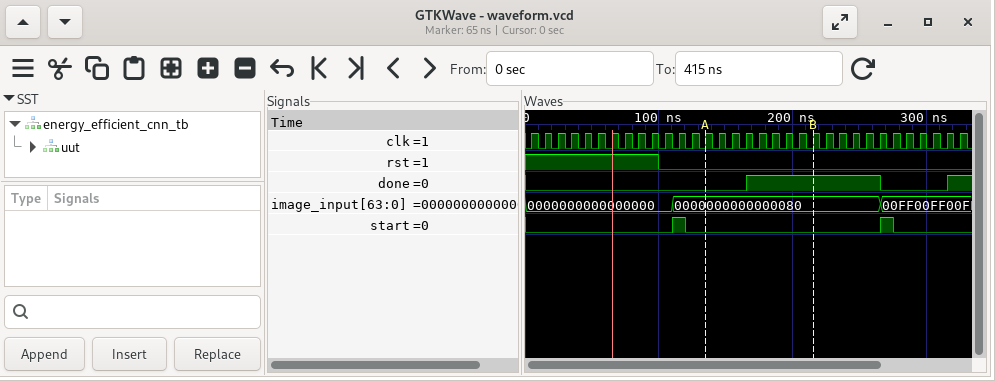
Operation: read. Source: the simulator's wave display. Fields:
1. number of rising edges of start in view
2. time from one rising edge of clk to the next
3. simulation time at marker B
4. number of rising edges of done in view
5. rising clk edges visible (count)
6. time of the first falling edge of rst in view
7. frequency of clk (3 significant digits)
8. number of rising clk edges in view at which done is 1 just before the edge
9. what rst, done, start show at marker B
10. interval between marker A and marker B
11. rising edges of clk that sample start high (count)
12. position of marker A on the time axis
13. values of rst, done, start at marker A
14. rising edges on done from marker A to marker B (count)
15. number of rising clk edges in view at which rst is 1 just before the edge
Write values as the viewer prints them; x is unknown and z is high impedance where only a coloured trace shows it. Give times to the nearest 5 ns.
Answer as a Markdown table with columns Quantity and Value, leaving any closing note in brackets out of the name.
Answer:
| Quantity | Value |
|---|---|
| number of rising edges of start in view | 2 |
| time from one rising edge of clk to the next | 10 ns |
| simulation time at marker B | 215 ns |
| number of rising edges of done in view | 2 |
| rising clk edges visible | 33 |
| time of the first falling edge of rst in view | 100 ns |
| frequency of clk | 100 MHz |
| number of rising clk edges in view at which done is 1 just before the edge | 11 |
| what rst, done, start show at marker B | rst=0, done=1, start=0 |
| interval between marker A and marker B | 80 ns |
| rising edges of clk that sample start high | 2 |
| position of marker A on the time axis | 135 ns |
| values of rst, done, start at marker A | rst=0, done=0, start=0 |
| rising edges on done from marker A to marker B | 1 |
| number of rising clk edges in view at which rst is 1 just before the edge | 10 |
